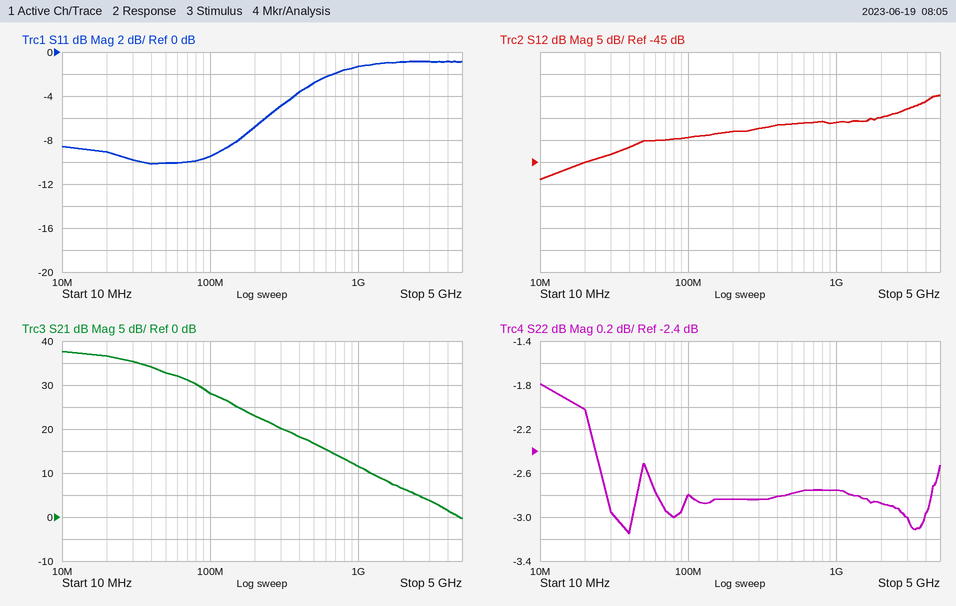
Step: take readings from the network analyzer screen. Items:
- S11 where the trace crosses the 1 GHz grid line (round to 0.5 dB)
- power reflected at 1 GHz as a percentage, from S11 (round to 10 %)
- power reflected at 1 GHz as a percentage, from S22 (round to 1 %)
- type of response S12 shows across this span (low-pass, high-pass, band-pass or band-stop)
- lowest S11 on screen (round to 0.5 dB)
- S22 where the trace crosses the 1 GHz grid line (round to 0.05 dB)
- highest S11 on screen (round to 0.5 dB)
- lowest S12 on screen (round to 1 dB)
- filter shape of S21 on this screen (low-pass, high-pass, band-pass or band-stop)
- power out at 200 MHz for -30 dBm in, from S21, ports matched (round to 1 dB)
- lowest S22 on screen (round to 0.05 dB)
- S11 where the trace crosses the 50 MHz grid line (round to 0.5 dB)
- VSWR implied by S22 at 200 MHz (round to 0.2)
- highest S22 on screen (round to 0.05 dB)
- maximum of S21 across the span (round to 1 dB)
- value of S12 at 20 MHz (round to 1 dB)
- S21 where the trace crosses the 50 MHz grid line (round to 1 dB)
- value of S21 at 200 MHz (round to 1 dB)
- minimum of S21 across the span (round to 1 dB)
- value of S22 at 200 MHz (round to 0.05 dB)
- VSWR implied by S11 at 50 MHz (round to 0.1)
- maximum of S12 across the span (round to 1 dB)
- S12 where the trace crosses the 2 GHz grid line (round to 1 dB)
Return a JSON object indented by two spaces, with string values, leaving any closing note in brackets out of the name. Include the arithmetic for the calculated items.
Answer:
{
  "S11 where the trace crosses the 1 GHz grid line": "-1.5 dB",
  "power reflected at 1 GHz as a percentage, from S11": "10^(-1.5/10) ≈ 70.8 %, so 70 % to the nearest 10 %",
  "power reflected at 1 GHz as a percentage, from S22": "10^(-2.75/10) ≈ 53 %",
  "type of response S12 shows across this span": "high-pass",
  "lowest S11 on screen": "-10.0 dB",
  "S22 where the trace crosses the 1 GHz grid line": "-2.75 dB",
  "highest S11 on screen": "-1.0 dB",
  "lowest S12 on screen": "-49 dB",
  "filter shape of S21 on this screen": "low-pass",
  "power out at 200 MHz for -30 dBm in, from S21, ports matched": "-30 dBm + (23 dB) = -7 dBm",
  "lowest S22 on screen": "-3.15 dB",
  "S11 where the trace crosses the 50 MHz grid line": "-10.0 dB",
  "VSWR implied by S22 at 200 MHz": "|Γ| = 10^(-2.85/20) = 0.7203; VSWR = (1 + 0.7203)/(1 − 0.7203) ≈ 6.2",
  "highest S22 on screen": "-1.80 dB",
  "maximum of S21 across the span": "38 dB",
  "value of S12 at 20 MHz": "-45 dB",
  "S21 where the trace crosses the 50 MHz grid line": "33 dB",
  "value of S21 at 200 MHz": "23 dB",
  "minimum of S21 across the span": "0 dB",
  "value of S22 at 200 MHz": "-2.85 dB",
  "VSWR implied by S11 at 50 MHz": "|Γ| = 10^(-10/20) = 0.3162; VSWR = (1 + 0.3162)/(1 − 0.3162) ≈ 1.9",
  "maximum of S12 across the span": "-30 dB",
  "S12 where the trace crosses the 2 GHz grid line": "-35 dB"
}
